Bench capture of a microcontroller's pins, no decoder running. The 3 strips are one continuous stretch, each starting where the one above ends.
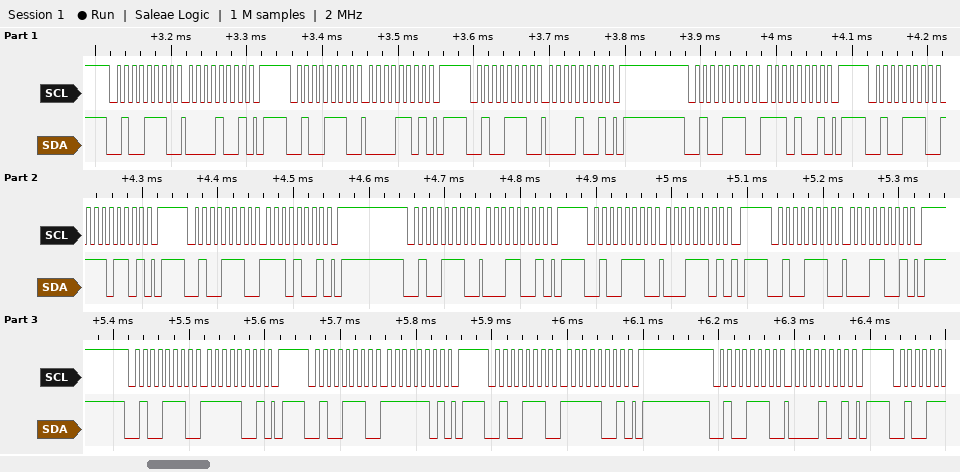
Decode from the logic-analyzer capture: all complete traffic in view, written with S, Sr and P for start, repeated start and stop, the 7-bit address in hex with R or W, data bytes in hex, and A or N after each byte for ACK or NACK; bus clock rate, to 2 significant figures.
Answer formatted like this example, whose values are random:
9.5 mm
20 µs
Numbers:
S 27W A 09 A P S 27W A 0D A P S 27W A 09 A P S 27W A E9 A P S 27W A ED A P S 27W A E9 A P S 27W A 19 A P S 27W A 1D A P S 27W A 19 A P S 27W A F9 A P S 27W A FD A P S 27W A F9 A P S 27W A 09 A P
100 kHz
